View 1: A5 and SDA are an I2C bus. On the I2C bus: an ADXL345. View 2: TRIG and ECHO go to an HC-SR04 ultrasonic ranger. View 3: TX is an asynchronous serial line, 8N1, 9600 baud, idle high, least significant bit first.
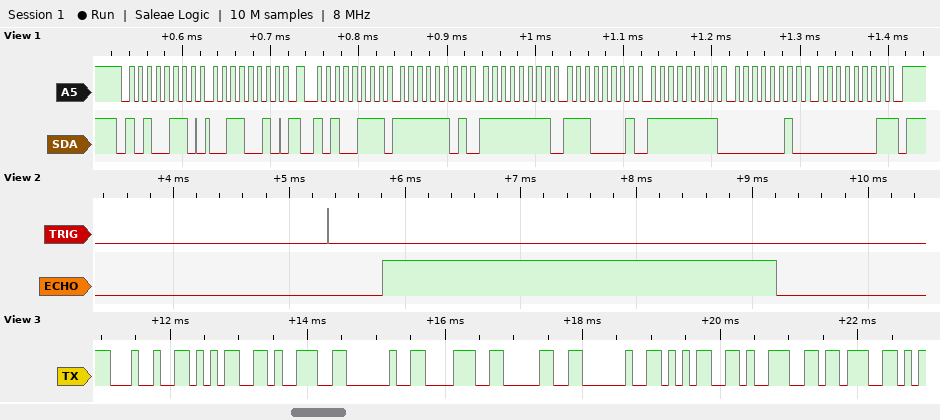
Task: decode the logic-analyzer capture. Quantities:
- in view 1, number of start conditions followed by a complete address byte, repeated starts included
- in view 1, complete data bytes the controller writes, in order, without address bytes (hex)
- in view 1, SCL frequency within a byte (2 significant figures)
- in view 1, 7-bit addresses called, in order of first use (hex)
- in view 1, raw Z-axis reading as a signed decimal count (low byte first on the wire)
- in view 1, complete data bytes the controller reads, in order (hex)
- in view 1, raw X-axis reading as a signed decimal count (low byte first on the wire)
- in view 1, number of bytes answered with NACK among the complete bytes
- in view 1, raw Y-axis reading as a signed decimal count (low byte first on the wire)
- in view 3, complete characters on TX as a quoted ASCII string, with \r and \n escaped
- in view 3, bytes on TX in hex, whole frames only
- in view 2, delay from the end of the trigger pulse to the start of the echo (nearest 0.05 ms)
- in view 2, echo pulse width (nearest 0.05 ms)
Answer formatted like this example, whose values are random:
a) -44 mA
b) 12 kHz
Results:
a) 2
b) 32
c) 100 kHz
d) 0x53
e) 258
f) FD FF E1 FF 02 01
g) -3
h) 1
i) -31
j) "$59 80 59;"
k) 24 35 39 20 38 30 20 35 39 3B
l) 0.45 ms
m) 3.40 ms
